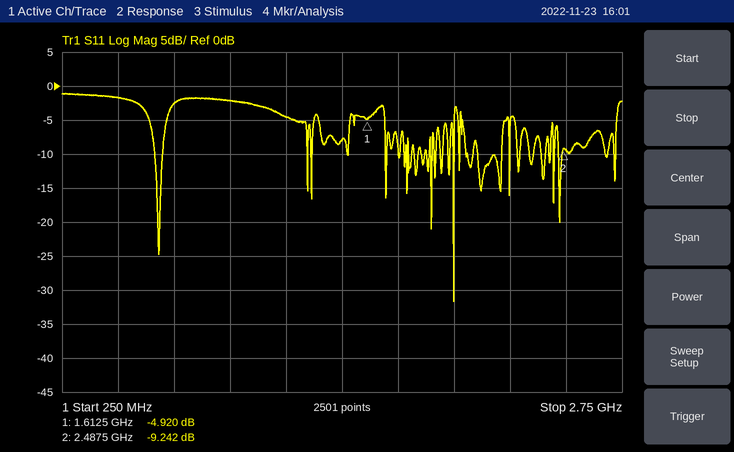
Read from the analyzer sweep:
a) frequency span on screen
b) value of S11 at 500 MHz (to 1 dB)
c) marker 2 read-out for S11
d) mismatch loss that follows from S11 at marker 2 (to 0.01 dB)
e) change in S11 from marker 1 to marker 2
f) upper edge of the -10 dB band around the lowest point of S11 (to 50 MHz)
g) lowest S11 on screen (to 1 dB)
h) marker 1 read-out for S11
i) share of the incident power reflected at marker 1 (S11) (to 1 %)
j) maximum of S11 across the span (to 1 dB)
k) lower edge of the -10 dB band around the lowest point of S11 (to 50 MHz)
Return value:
2.5 GHz
-2 dB
-9.242 dB
0.55 dB
-4.322 dB
2.00 GHz
-32 dB
-4.920 dB
32 %
-1 dB
2.00 GHz
